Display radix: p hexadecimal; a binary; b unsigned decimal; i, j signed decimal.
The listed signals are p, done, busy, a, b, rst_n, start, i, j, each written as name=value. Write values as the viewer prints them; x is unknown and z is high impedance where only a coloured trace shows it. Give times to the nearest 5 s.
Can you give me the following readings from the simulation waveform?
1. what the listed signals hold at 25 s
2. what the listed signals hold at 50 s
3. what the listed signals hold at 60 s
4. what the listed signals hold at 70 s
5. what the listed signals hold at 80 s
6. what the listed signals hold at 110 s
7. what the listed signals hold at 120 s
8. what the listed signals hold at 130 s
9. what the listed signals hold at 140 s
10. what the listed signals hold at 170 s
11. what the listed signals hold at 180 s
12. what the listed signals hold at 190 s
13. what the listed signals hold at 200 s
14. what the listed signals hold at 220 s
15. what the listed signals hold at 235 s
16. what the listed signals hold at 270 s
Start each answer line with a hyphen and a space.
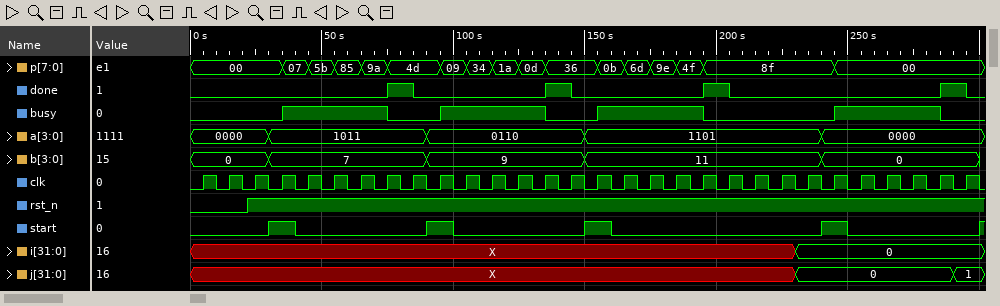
- p=00, done=0, busy=0, a=0000, b=0, rst_n=1, start=0, i=X, j=X
- p=5b, done=0, busy=1, a=1011, b=7, rst_n=1, start=0, i=X, j=X
- p=85, done=0, busy=1, a=1011, b=7, rst_n=1, start=0, i=X, j=X
- p=9a, done=0, busy=1, a=1011, b=7, rst_n=1, start=0, i=X, j=X
- p=4d, done=1, busy=0, a=1011, b=7, rst_n=1, start=0, i=X, j=X
- p=34, done=0, busy=1, a=0110, b=9, rst_n=1, start=0, i=X, j=X
- p=1a, done=0, busy=1, a=0110, b=9, rst_n=1, start=0, i=X, j=X
- p=0d, done=0, busy=1, a=0110, b=9, rst_n=1, start=0, i=X, j=X
- p=36, done=1, busy=0, a=0110, b=9, rst_n=1, start=0, i=X, j=X
- p=6d, done=0, busy=1, a=1101, b=11, rst_n=1, start=0, i=X, j=X
- p=9e, done=0, busy=1, a=1101, b=11, rst_n=1, start=0, i=X, j=X
- p=4f, done=0, busy=1, a=1101, b=11, rst_n=1, start=0, i=X, j=X
- p=8f, done=1, busy=0, a=1101, b=11, rst_n=1, start=0, i=X, j=X
- p=8f, done=0, busy=0, a=1101, b=11, rst_n=1, start=0, i=X, j=X
- p=8f, done=0, busy=0, a=1101, b=11, rst_n=1, start=0, i=0, j=0
- p=00, done=0, busy=1, a=0000, b=0, rst_n=1, start=0, i=0, j=0
